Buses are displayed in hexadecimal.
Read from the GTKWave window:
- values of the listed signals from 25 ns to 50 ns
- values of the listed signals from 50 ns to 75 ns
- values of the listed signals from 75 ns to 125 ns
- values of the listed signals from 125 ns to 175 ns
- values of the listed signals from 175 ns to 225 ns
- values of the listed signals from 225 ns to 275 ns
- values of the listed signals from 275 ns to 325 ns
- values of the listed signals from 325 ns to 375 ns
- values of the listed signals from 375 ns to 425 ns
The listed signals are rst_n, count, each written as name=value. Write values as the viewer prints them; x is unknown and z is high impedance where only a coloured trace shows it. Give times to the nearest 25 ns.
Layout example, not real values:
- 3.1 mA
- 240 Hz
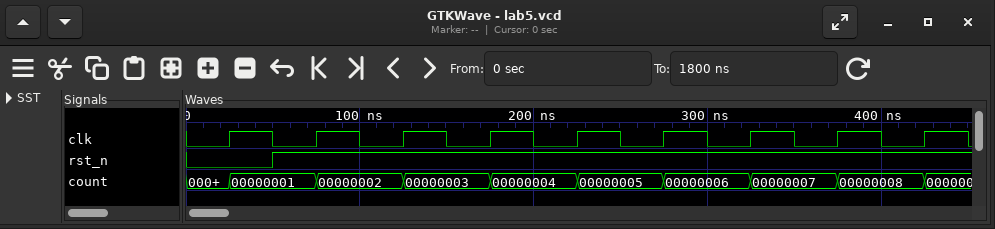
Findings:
- rst_n=0, count=00000001
- rst_n=1, count=00000001
- rst_n=1, count=00000002
- rst_n=1, count=00000003
- rst_n=1, count=00000004
- rst_n=1, count=00000005
- rst_n=1, count=00000006
- rst_n=1, count=00000007
- rst_n=1, count=00000008
